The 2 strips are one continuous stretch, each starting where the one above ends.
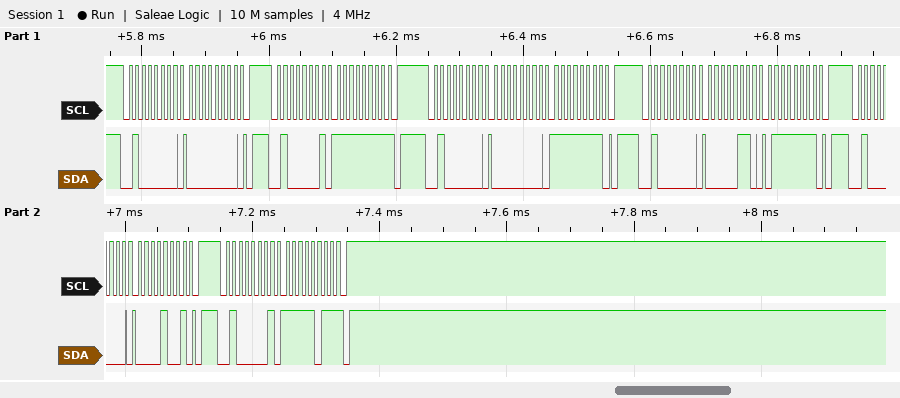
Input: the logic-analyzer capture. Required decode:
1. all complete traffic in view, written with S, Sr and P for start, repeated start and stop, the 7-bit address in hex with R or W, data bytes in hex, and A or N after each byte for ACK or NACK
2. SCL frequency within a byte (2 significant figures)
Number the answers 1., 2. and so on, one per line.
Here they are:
1. S 20W A 00 A P S 20R A FF N P S 20W A 00 A FF A P S 20W A 06 A 7F A P S 20W A 09 A P S 20R A FB N P
2. 100 kHz
